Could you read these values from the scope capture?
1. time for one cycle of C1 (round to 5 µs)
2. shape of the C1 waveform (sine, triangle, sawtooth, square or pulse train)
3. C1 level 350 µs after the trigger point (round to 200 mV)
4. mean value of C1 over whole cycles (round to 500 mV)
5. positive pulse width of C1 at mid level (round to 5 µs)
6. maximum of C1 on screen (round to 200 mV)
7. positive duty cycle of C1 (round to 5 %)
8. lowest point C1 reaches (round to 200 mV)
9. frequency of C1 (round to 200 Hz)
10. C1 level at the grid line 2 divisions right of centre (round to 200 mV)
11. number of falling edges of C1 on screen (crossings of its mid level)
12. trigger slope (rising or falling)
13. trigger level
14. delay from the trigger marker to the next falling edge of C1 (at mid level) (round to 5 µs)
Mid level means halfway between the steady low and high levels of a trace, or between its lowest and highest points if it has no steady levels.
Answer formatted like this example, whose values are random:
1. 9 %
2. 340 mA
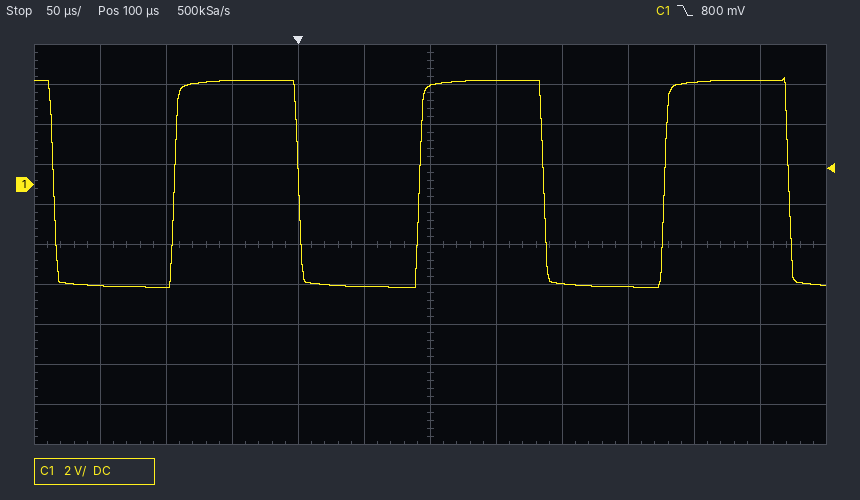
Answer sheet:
1. 185 µs
2. square
3. 5.2 V
4. 0.0 V
5. 95 µs
6. 5.4 V
7. 50 %
8. -5.2 V
9. 5.4 kHz
10. -5.0 V
11. 4
12. falling
13. 800 mV
14. 185 µs
